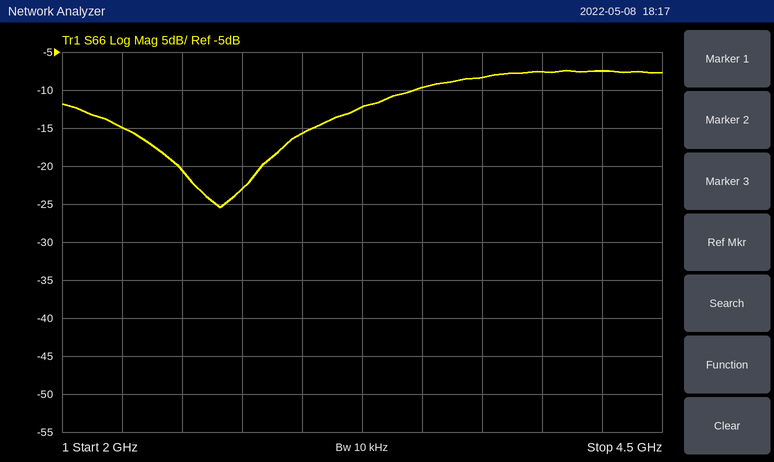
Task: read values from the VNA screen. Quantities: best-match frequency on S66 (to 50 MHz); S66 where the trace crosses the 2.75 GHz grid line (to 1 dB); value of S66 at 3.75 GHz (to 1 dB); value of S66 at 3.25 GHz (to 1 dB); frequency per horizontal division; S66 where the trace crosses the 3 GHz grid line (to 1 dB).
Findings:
2.65 GHz
-23 dB
-8 dB
-12 dB
250 MHz
-16 dB
